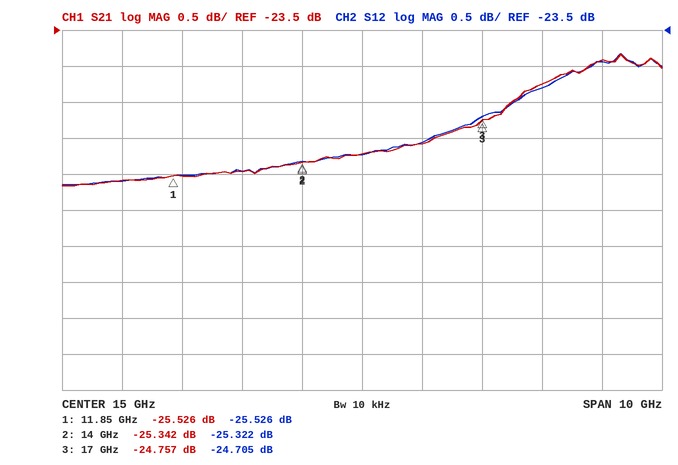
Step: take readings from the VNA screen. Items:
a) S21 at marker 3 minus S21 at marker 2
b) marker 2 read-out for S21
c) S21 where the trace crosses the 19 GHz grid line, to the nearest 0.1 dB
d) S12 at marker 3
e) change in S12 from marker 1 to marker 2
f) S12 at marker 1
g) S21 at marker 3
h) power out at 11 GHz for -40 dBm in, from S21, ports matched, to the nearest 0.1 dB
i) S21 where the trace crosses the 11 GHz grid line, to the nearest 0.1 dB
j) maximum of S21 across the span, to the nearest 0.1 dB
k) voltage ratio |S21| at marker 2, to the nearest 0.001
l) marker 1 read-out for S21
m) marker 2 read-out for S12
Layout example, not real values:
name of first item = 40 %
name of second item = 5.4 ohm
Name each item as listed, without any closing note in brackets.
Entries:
S21 at marker 3 minus S21 at marker 2 = 0.585 dB
marker 2 read-out for S21 = -25.342 dB
S21 where the trace crosses the 19 GHz grid line, to the nearest 0.1 dB = -23.9 dB
S12 at marker 3 = -24.705 dB
change in S12 from marker 1 to marker 2 = 0.204 dB
S12 at marker 1 = -25.526 dB
S21 at marker 3 = -24.757 dB
power out at 11 GHz for -40 dBm in, from S21, ports matched, to the nearest 0.1 dB = -65.6 dBm
S21 where the trace crosses the 11 GHz grid line, to the nearest 0.1 dB = -25.6 dB
maximum of S21 across the span, to the nearest 0.1 dB = -23.8 dB
voltage ratio |S21| at marker 2, to the nearest 0.001 = 0.054
marker 1 read-out for S21 = -25.526 dB
marker 2 read-out for S12 = -25.322 dB
